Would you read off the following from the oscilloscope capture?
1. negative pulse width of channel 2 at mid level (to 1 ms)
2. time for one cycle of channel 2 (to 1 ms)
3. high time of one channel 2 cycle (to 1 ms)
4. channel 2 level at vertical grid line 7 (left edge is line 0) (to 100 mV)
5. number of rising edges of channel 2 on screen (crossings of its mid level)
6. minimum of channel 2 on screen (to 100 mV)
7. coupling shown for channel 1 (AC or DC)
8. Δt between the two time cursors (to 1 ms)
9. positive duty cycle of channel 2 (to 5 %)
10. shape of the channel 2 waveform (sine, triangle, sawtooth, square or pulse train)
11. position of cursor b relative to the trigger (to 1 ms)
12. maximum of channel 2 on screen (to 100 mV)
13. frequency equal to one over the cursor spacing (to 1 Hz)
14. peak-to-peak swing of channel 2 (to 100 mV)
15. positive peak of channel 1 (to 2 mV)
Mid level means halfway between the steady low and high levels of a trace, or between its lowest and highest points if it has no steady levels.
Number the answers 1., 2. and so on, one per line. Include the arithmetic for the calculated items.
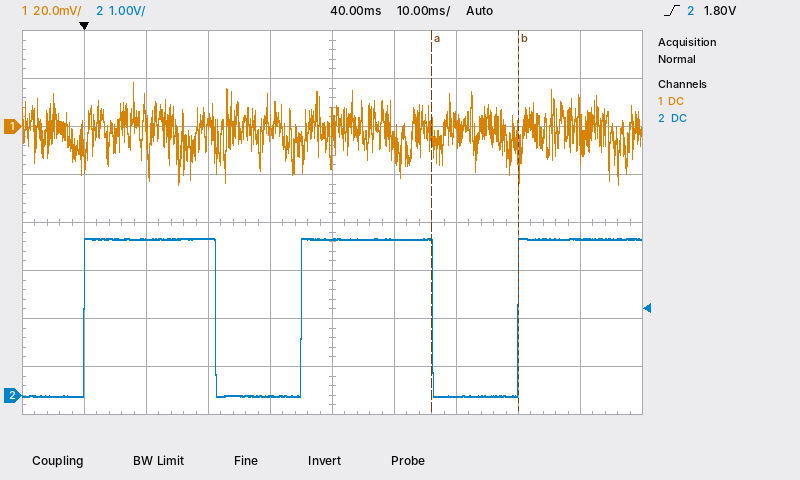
1. 14 ms
2. 35 ms
3. 21 ms
4. 0.0 V
5. 3
6. 0.0 V
7. DC
8. 14 ms
9. 21 ms / 35 ms ≈ 60 %
10. pulse train
11. +70 ms
12. 3.3 V
13. 1 / 14 ms ≈ 71 Hz
14. 3.3 V − (0.0 V) = 3.3 V
15. 18 mV
